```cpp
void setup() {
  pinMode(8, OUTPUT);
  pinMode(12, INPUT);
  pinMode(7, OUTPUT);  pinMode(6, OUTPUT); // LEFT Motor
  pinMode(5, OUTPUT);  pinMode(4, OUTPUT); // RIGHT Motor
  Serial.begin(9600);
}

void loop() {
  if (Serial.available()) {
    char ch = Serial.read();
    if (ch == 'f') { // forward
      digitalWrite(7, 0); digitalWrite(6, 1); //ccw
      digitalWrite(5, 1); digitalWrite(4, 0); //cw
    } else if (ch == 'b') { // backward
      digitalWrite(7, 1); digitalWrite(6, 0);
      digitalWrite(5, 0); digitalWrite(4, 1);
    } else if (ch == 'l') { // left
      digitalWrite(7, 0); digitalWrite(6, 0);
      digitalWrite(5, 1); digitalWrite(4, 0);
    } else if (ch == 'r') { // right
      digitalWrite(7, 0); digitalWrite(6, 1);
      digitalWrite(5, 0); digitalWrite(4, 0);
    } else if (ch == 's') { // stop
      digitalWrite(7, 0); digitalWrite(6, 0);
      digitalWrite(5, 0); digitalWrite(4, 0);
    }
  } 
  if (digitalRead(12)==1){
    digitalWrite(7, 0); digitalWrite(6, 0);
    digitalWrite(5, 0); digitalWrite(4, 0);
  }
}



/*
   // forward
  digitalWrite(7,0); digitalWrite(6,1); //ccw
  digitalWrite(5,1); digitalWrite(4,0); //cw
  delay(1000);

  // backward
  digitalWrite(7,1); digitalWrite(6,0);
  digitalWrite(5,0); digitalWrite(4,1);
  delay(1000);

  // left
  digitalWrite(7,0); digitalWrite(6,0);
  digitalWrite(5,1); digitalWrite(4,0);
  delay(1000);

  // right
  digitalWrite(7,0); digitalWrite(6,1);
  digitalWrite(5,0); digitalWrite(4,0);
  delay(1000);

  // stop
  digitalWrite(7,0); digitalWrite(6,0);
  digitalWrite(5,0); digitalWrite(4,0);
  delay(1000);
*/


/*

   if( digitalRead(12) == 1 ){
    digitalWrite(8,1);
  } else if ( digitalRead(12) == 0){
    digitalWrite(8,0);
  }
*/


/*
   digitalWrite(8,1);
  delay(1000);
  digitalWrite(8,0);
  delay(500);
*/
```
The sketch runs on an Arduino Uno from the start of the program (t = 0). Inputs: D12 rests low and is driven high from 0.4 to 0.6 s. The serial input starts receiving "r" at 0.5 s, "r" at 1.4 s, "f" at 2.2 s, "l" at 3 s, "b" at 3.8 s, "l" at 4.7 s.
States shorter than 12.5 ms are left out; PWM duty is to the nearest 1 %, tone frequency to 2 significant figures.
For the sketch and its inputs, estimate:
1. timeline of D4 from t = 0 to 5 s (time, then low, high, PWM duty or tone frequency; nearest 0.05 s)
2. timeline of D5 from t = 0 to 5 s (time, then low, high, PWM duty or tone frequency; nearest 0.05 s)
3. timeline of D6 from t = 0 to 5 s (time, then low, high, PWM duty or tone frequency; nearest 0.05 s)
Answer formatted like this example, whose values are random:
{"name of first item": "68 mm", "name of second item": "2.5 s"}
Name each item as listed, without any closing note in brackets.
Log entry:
{"timeline of D4 from t = 0 to 5 s": "0 s low; 3.8 s high; 4.7 s low", "timeline of D5 from t = 0 to 5 s": "0 s low; 2.2 s high; 3.8 s low; 4.7 s high", "timeline of D6 from t = 0 to 5 s": "0 s low; 1.4 s high; 3 s low"}
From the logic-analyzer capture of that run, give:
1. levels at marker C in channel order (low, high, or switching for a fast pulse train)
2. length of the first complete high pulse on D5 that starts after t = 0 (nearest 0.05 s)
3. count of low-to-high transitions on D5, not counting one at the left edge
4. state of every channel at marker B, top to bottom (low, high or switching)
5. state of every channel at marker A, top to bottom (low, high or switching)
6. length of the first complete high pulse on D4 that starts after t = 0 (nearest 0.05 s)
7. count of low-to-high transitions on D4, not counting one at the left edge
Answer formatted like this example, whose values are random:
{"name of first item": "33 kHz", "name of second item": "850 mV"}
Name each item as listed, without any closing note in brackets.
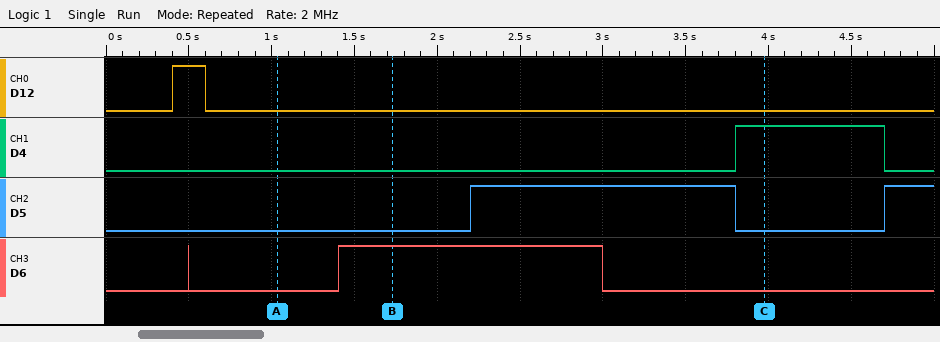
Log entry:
{"levels at marker C in channel order": "D12 low, D4 high, D5 low, D6 low", "length of the first complete high pulse on D5 that starts after t = 0": "1.60 s", "count of low-to-high transitions on D5, not counting one at the left edge": "2", "state of every channel at marker B, top to bottom": "D12 low, D4 low, D5 low, D6 high", "state of every channel at marker A, top to bottom": "D12 low, D4 low, D5 low, D6 low", "length of the first complete high pulse on D4 that starts after t = 0": "0.90 s", "count of low-to-high transitions on D4, not counting one at the left edge": "1"}
